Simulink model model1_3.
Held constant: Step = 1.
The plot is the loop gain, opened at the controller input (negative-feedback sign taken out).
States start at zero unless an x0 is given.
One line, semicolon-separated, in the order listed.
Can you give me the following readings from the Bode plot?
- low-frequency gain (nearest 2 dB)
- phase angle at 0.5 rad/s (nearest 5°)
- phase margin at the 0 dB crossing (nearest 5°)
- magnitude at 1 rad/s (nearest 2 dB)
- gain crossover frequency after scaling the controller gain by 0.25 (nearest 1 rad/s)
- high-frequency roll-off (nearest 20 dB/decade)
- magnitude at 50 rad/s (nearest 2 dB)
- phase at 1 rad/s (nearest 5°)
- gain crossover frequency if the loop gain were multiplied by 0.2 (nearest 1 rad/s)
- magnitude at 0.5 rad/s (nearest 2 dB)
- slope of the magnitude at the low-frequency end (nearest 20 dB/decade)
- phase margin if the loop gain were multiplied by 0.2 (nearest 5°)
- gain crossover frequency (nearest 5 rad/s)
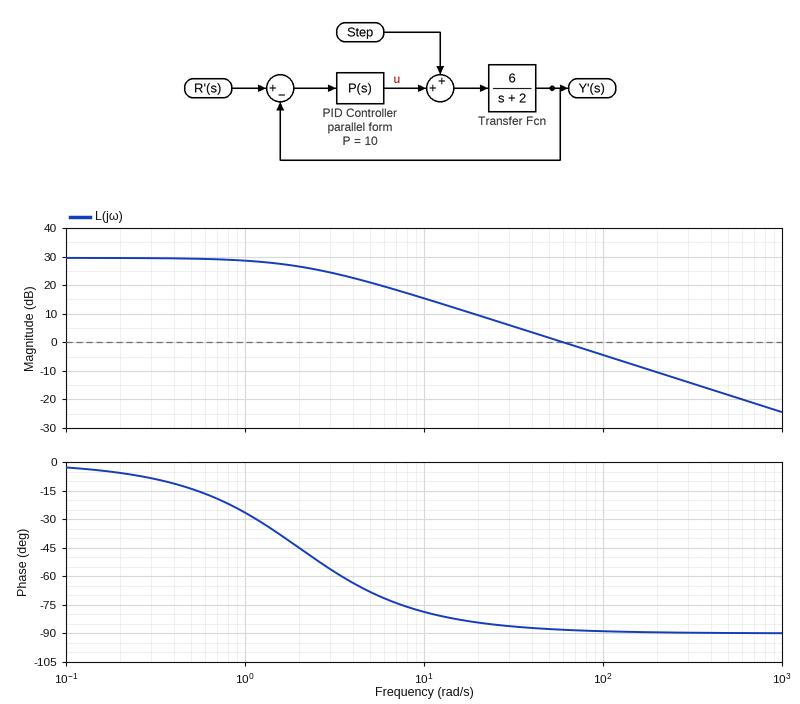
30 dB; -15°; 90°; 28 dB; 15 rad/s; -20 dB/decade; 2 dB; -25°; 12 rad/s; 30 dB; 0 dB/decade; 100°; 60 rad/s
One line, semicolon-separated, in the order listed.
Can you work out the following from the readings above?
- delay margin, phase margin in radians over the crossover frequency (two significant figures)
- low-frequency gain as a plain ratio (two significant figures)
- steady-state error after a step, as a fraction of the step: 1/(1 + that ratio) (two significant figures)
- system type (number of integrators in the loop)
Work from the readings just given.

0.026 s; 32; 0.030; 0
